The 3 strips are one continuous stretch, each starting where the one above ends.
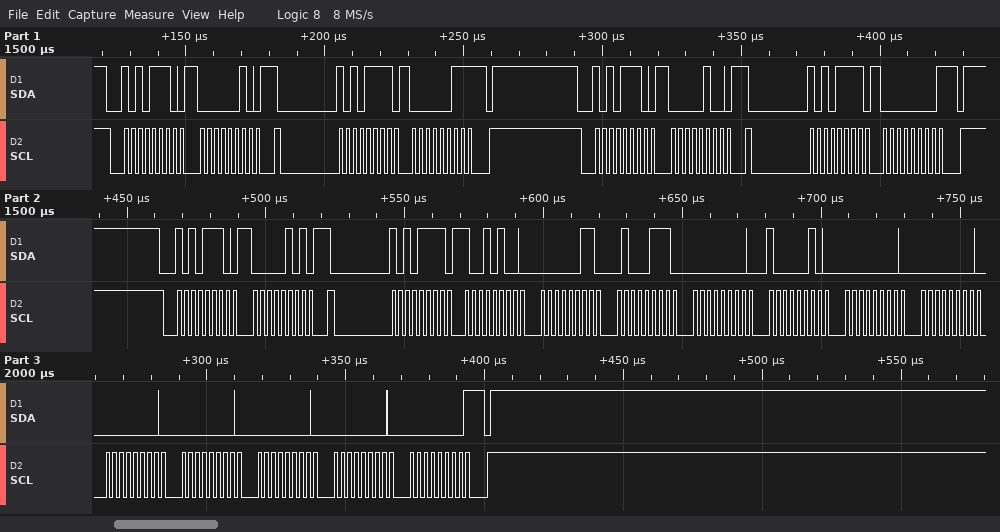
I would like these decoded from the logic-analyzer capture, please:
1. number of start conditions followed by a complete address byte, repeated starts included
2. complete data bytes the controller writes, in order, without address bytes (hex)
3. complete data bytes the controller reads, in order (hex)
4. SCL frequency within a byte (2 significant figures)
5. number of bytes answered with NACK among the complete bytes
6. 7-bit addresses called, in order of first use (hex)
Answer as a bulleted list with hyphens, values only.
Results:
- 6
- 02 04 05
- 03 00 94 03 47 00 82 00 00 00 00 00 00 00
- 400 kHz
- 3
- 0x57
